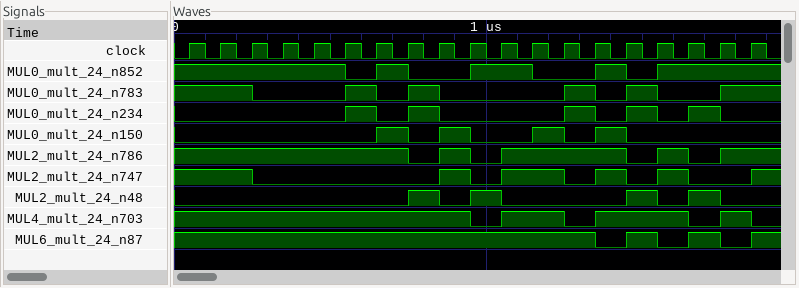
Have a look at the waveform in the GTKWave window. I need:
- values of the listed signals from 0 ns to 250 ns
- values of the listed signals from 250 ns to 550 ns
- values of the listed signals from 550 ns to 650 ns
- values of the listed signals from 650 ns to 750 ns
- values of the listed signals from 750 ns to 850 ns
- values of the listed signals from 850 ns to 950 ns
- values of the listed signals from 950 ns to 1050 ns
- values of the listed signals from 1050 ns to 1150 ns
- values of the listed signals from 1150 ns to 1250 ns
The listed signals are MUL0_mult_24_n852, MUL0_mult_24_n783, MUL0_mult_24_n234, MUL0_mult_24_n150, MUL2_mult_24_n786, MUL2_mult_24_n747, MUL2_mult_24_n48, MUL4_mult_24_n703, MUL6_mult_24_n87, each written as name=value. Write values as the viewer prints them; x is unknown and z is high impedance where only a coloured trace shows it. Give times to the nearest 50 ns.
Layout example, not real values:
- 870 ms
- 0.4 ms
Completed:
- MUL0_mult_24_n852=1, MUL0_mult_24_n783=1, MUL0_mult_24_n234=0, MUL0_mult_24_n150=0, MUL2_mult_24_n786=1, MUL2_mult_24_n747=1, MUL2_mult_24_n48=0, MUL4_mult_24_n703=1, MUL6_mult_24_n87=1
- MUL0_mult_24_n852=1, MUL0_mult_24_n783=0, MUL0_mult_24_n234=0, MUL0_mult_24_n150=0, MUL2_mult_24_n786=1, MUL2_mult_24_n747=0, MUL2_mult_24_n48=0, MUL4_mult_24_n703=1, MUL6_mult_24_n87=1
- MUL0_mult_24_n852=0, MUL0_mult_24_n783=1, MUL0_mult_24_n234=1, MUL0_mult_24_n150=0, MUL2_mult_24_n786=1, MUL2_mult_24_n747=0, MUL2_mult_24_n48=0, MUL4_mult_24_n703=1, MUL6_mult_24_n87=1
- MUL0_mult_24_n852=1, MUL0_mult_24_n783=0, MUL0_mult_24_n234=0, MUL0_mult_24_n150=1, MUL2_mult_24_n786=1, MUL2_mult_24_n747=0, MUL2_mult_24_n48=0, MUL4_mult_24_n703=1, MUL6_mult_24_n87=1
- MUL0_mult_24_n852=0, MUL0_mult_24_n783=1, MUL0_mult_24_n234=1, MUL0_mult_24_n150=0, MUL2_mult_24_n786=0, MUL2_mult_24_n747=0, MUL2_mult_24_n48=1, MUL4_mult_24_n703=1, MUL6_mult_24_n87=1
- MUL0_mult_24_n852=0, MUL0_mult_24_n783=0, MUL0_mult_24_n234=0, MUL0_mult_24_n150=1, MUL2_mult_24_n786=1, MUL2_mult_24_n747=1, MUL2_mult_24_n48=0, MUL4_mult_24_n703=1, MUL6_mult_24_n87=1
- MUL0_mult_24_n852=1, MUL0_mult_24_n783=0, MUL0_mult_24_n234=0, MUL0_mult_24_n150=0, MUL2_mult_24_n786=0, MUL2_mult_24_n747=0, MUL2_mult_24_n48=1, MUL4_mult_24_n703=0, MUL6_mult_24_n87=1
- MUL0_mult_24_n852=1, MUL0_mult_24_n783=0, MUL0_mult_24_n234=0, MUL0_mult_24_n150=0, MUL2_mult_24_n786=1, MUL2_mult_24_n747=1, MUL2_mult_24_n48=0, MUL4_mult_24_n703=1, MUL6_mult_24_n87=1
- MUL0_mult_24_n852=0, MUL0_mult_24_n783=0, MUL0_mult_24_n234=0, MUL0_mult_24_n150=1, MUL2_mult_24_n786=1, MUL2_mult_24_n747=1, MUL2_mult_24_n48=0, MUL4_mult_24_n703=1, MUL6_mult_24_n87=1
